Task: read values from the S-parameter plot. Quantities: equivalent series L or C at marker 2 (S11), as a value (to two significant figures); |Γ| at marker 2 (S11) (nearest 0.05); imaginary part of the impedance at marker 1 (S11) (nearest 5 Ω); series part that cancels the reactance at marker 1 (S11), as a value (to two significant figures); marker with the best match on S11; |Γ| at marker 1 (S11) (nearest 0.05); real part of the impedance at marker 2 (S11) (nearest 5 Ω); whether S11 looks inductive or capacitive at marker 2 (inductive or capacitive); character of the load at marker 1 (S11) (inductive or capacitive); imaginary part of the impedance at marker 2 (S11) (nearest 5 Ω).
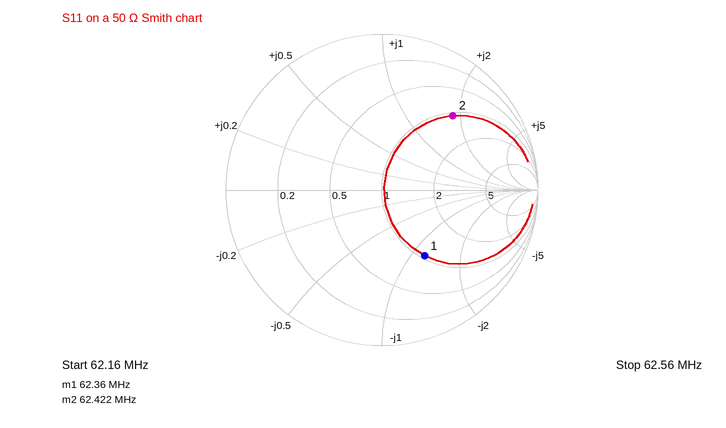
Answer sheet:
230 nH
0.65
-60 Ω
150 nH
marker 1
0.50
55 Ω
inductive
capacitive
+90 Ω
